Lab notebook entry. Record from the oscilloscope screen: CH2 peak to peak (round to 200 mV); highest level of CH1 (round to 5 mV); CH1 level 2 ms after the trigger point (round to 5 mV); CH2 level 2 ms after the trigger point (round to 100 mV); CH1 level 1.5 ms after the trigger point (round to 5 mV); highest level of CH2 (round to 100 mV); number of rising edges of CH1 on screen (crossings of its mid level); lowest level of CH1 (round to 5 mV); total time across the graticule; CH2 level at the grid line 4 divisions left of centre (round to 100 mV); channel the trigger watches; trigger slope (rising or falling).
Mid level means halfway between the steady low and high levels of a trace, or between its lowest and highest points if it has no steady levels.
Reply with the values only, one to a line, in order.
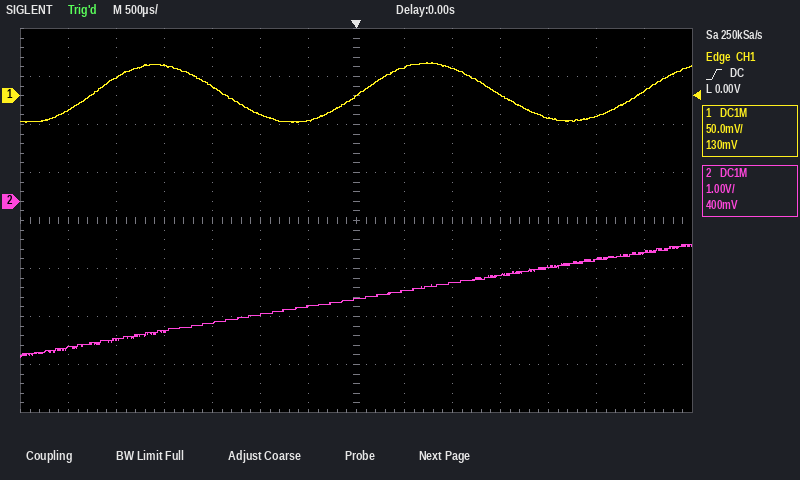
2.4 V
35 mV
-25 mV
-1.4 V
0 mV
-900 mV
3
-30 mV
7 ms
-2.7 V
CH1
rising
